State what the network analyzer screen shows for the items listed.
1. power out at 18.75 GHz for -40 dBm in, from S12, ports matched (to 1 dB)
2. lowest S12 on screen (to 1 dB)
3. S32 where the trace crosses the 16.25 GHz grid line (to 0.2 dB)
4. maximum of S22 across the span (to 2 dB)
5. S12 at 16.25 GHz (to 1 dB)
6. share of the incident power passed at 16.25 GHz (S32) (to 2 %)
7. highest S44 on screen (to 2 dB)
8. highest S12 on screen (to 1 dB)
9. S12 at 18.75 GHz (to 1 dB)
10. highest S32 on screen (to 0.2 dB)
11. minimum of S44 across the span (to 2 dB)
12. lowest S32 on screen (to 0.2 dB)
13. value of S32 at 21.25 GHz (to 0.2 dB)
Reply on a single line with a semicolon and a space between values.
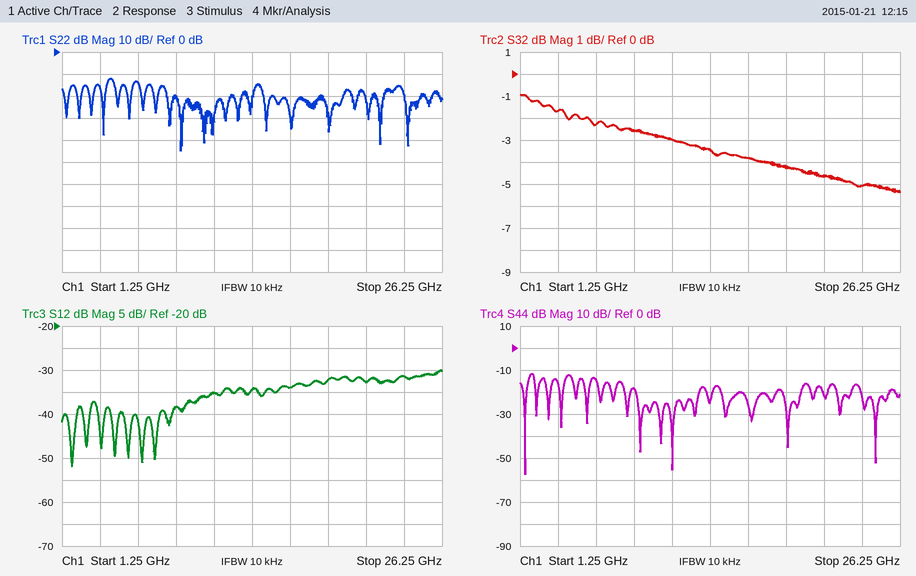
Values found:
-72 dBm; -52 dB; -3.8 dB; -12 dB; -34 dB; 42 %; -12 dB; -30 dB; -32 dB; -1.0 dB; -58 dB; -5.4 dB; -4.6 dB
